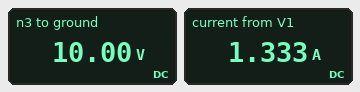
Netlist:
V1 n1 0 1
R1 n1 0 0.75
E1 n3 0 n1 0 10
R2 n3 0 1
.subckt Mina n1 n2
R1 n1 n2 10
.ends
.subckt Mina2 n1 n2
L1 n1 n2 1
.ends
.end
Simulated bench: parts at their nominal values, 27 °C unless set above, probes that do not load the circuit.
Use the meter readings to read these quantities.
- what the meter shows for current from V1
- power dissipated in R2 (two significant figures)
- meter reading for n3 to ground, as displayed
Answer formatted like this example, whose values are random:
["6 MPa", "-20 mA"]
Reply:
["1.333 A", "100 W", "10.00 V"]
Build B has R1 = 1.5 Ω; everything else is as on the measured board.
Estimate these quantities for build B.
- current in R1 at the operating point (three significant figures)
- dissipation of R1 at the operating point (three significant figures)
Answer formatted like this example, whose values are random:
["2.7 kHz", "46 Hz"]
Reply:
["667 mA", "667 mW"]
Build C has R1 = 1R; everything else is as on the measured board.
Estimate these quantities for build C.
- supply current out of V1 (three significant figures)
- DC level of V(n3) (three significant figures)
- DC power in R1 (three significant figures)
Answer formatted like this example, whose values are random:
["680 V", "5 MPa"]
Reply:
["1.00 A", "10.0 V", "1.00 W"]
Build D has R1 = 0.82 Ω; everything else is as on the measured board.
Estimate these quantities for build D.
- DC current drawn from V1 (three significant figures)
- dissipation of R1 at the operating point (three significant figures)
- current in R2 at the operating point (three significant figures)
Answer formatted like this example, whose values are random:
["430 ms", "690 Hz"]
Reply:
["1.22 A", "1.22 W", "10.0 A"]
